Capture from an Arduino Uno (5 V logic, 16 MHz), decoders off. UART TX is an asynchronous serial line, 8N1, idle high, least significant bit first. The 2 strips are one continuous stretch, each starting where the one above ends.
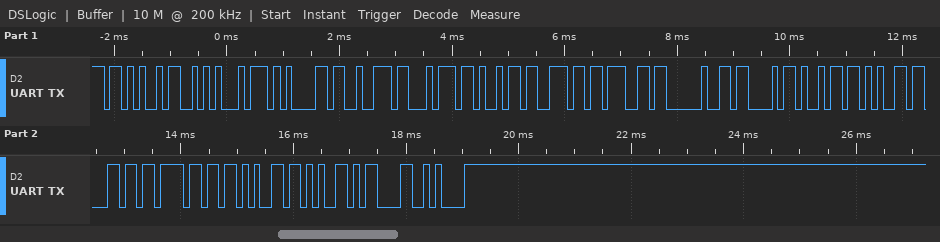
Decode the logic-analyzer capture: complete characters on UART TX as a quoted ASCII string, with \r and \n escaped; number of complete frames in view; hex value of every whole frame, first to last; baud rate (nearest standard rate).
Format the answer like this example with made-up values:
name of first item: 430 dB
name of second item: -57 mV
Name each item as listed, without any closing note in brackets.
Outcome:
complete characters on UART TX as a quoted ASCII string, with \r and \n escaped: "+Starting Cielo++\r\n"
number of complete frames in view: 19
hex value of every whole frame, first to last: 2B 53 74 61 72 74 69 6E 67 20 43 69 65 6C 6F 2B 2B 0D 0A
baud rate: 9600 baud
